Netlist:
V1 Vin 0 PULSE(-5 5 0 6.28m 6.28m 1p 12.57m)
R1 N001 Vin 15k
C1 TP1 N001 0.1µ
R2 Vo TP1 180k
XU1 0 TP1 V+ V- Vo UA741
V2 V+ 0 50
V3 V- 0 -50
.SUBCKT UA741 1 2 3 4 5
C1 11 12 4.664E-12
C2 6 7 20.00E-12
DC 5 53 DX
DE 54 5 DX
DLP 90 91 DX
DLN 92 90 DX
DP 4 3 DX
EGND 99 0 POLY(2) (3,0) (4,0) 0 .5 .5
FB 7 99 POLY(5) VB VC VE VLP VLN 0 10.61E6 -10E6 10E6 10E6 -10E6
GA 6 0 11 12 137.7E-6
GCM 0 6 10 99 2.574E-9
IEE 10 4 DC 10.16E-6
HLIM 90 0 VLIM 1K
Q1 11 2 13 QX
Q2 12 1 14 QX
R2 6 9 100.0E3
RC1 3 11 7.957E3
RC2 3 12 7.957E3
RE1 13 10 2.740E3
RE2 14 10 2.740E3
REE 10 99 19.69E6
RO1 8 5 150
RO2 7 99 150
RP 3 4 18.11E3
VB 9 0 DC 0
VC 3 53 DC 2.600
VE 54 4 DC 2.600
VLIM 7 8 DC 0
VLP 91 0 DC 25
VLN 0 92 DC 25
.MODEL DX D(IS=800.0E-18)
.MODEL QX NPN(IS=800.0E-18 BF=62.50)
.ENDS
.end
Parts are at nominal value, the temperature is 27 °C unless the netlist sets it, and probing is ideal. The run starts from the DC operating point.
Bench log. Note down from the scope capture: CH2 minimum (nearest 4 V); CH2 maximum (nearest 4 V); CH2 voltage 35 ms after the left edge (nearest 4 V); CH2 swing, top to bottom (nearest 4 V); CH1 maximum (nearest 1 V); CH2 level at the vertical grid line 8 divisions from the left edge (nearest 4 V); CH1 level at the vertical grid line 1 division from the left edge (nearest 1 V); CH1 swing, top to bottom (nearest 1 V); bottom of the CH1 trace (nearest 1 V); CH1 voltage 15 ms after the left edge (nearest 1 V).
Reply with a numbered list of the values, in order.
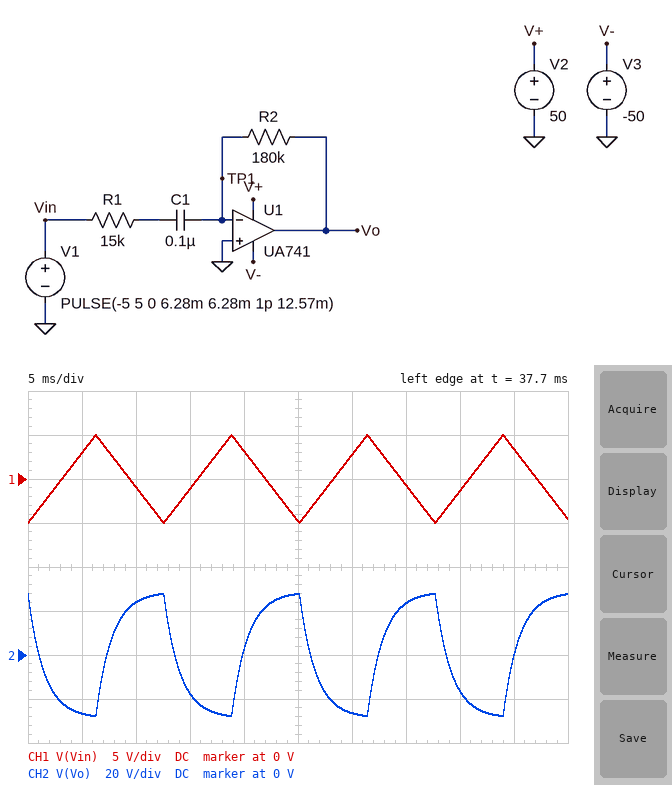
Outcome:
1. -28 V
2. 28 V
3. 24 V
4. 56 V
5. 5 V
6. -16 V
7. 3 V
8. 10 V
9. -5 V
10. -1 V
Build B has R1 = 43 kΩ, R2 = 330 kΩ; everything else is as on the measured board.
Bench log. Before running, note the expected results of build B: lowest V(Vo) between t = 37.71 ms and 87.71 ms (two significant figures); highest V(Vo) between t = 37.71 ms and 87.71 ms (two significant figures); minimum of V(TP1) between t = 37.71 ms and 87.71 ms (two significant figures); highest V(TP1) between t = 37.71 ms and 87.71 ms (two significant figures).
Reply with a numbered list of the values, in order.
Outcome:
1. -33 V
2. 33 V
3. -2.7 mV
4. 2.7 mV
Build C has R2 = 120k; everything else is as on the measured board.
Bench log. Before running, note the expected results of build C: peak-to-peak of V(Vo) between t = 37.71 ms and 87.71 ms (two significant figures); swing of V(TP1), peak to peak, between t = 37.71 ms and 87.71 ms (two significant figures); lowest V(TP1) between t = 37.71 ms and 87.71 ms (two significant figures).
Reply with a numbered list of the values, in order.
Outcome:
1. 37 V
2. 7.1 mV
3. -3.5 mV
